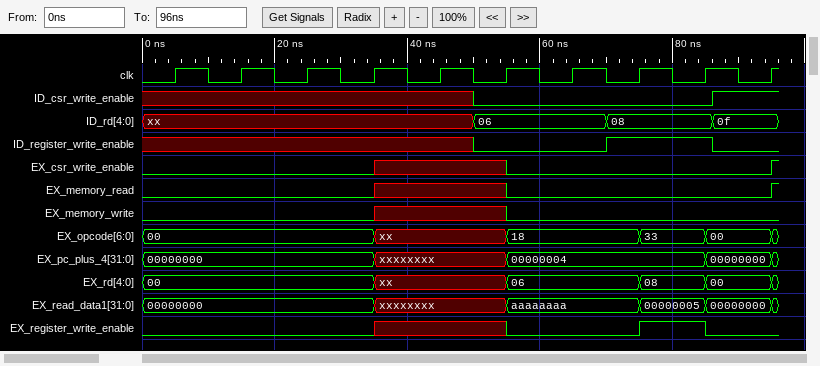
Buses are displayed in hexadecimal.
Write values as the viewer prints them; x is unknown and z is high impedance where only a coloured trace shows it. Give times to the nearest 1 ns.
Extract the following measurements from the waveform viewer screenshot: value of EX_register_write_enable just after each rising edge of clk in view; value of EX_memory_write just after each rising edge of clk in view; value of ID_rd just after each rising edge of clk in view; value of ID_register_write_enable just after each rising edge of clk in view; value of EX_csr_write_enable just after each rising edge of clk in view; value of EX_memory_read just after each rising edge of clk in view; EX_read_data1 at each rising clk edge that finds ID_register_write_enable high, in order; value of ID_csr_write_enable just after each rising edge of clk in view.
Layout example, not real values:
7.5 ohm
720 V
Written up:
0 0 0 x x 0 0 1 0 0
0 0 0 x x 0 0 0 0 0
xx, xx, xx, xx, xx, 06, 06, 08, 08, 0f
x x x x x 0 0 1 1 0
0 0 0 x x 0 0 0 0 1
0 0 0 x x 0 0 0 0 1
aaaaaaaa, 00000005
x x x x x 0 0 0 0 1
